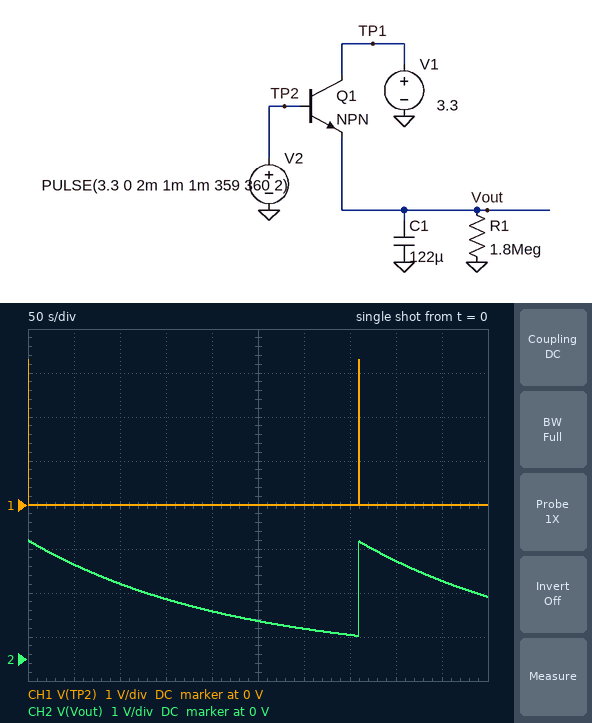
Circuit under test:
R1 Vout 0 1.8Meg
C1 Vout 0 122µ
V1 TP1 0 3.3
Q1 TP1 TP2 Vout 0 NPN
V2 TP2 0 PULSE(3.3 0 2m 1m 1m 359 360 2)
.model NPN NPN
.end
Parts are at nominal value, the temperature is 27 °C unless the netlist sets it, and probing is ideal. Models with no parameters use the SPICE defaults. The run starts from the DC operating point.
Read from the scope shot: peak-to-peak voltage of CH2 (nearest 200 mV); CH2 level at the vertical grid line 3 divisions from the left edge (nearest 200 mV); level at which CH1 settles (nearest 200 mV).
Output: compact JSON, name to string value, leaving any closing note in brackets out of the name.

{"peak-to-peak voltage of CH2": "2.2 V", "CH2 level at the vertical grid line 3 divisions from the left edge": "1.4 V", "level at which CH1 settles": "0 V"}
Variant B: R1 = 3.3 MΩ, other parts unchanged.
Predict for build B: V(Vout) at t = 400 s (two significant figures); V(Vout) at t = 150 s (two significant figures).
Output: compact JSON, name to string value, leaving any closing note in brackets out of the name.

{"V(Vout) at t = 400 s": "2.4 V", "V(Vout) at t = 150 s": "1.9 V"}
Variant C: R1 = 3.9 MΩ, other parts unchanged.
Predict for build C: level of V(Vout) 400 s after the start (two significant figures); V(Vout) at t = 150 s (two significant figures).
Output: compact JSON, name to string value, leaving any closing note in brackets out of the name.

{"level of V(Vout) 400 s after the start": "2.5 V", "V(Vout) at t = 150 s": "2.0 V"}
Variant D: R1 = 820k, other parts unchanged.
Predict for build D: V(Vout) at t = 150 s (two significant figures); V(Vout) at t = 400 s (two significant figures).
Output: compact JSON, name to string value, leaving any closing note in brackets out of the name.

{"V(Vout) at t = 150 s": "600 mV", "V(Vout) at t = 400 s": "1.8 V"}
